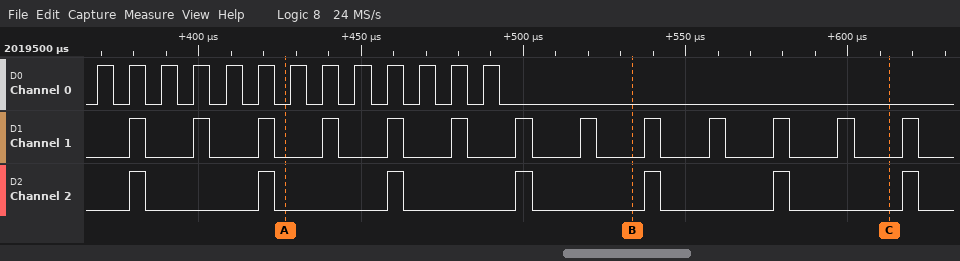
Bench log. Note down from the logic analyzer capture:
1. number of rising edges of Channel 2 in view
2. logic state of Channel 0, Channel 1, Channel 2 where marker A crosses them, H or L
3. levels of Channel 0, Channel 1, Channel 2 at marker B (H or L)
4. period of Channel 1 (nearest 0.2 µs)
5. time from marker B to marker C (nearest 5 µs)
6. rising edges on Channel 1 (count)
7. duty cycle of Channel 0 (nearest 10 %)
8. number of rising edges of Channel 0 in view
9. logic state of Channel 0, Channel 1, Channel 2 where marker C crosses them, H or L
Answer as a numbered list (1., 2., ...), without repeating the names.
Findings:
1. 7
2. Channel 0=L, Channel 1=L, Channel 2=L
3. Channel 0=L, Channel 1=L, Channel 2=L
4. 19.8 µs
5. 80 µs
6. 13
7. 50 %
8. 13
9. Channel 0=L, Channel 1=L, Channel 2=L
